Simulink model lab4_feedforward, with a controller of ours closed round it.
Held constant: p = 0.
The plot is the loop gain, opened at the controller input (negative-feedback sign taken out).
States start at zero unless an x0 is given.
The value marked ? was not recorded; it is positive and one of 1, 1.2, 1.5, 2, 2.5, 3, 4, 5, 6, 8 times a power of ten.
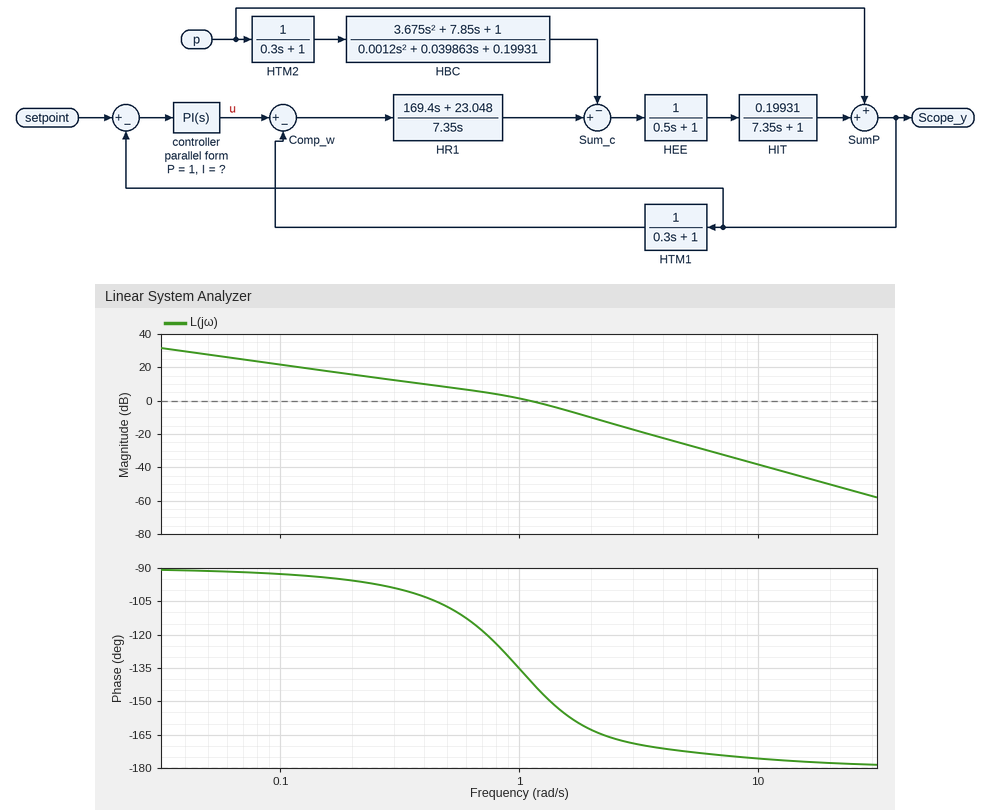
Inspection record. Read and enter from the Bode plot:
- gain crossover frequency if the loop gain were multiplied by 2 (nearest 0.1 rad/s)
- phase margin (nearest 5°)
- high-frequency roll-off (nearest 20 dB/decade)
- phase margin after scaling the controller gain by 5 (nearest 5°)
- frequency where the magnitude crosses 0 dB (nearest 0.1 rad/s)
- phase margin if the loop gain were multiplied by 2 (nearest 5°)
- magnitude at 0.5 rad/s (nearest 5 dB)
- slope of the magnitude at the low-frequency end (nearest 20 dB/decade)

1.6 rad/s
40°
-40 dB/decade
15°
1.1 rad/s
25°
10 dB
-20 dB/decade
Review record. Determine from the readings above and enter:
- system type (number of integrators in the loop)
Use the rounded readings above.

1
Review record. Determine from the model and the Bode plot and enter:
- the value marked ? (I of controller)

1.2
